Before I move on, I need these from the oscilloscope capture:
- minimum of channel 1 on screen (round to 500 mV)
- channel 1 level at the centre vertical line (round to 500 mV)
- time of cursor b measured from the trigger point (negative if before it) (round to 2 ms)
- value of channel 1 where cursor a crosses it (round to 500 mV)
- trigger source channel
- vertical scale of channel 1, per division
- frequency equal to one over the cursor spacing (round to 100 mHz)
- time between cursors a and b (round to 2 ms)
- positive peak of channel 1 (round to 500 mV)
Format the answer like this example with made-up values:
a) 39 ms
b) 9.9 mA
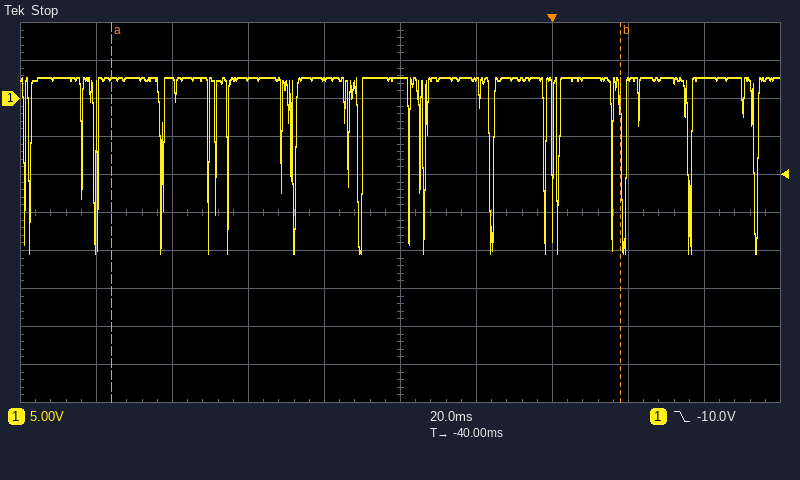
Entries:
a) -20.5 V
b) 3.0 V
c) +18 ms
d) 2.5 V
e) channel 1
f) 5 V
g) 7.5 Hz
h) 134 ms
i) 3.0 V
